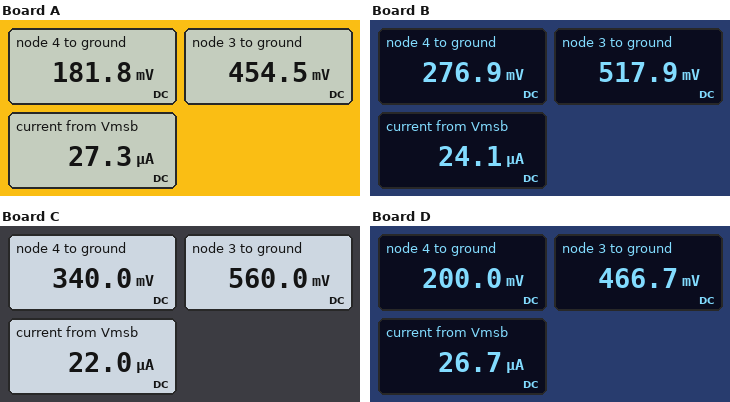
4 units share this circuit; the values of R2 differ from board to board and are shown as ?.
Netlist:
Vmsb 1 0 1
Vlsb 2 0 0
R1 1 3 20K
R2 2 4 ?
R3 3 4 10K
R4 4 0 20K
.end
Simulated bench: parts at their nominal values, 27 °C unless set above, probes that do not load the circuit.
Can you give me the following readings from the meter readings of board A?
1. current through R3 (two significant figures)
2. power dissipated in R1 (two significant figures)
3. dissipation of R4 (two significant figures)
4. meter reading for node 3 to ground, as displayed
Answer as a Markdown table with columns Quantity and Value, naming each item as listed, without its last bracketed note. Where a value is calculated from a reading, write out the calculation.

| Quantity | Value |
|---|---|
| current through R3 | (454.5 mV - 181.8 mV) / 10 kΩ = 27 µA |
| power dissipated in R1 | (1 V - 454.5 mV)^2 / 20 kΩ = 15 µW |
| dissipation of R4 | (181.8 mV)^2 / 20 kΩ = 1.7 µW |
| meter reading for node 3 to ground, as displayed | 454.5 mV |
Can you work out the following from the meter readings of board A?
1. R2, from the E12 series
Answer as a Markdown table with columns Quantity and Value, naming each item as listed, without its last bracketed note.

| Quantity | Value |
|---|---|
| R2, from the E12 series | 10 kΩ |
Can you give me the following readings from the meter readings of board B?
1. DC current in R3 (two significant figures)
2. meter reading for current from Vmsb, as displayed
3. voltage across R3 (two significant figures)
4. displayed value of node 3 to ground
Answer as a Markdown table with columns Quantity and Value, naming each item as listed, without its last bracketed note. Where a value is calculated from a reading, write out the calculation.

| Quantity | Value |
|---|---|
| DC current in R3 | (517.9 mV - 276.9 mV) / 10 kΩ = 24 µA |
| meter reading for current from Vmsb, as displayed | 24.1 µA |
| voltage across R3 | 517.9 mV - 276.9 mV = 240 mV |
| displayed value of node 3 to ground | 517.9 mV |
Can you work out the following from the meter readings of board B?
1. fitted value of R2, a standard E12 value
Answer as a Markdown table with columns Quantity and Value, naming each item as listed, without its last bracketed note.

| Quantity | Value |
|---|---|
| fitted value of R2, a standard E12 value | 27 kΩ |
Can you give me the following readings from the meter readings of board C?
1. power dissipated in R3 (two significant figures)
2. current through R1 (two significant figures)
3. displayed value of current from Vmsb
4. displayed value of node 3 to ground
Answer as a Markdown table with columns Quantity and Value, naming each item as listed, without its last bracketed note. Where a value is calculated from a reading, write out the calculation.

| Quantity | Value |
|---|---|
| power dissipated in R3 | (560 mV - 340 mV)^2 / 10 kΩ = 4.8 µW |
| current through R1 | (1 V - 560 mV) / 20 kΩ = 22 µA |
| displayed value of current from Vmsb | 22.0 µA |
| displayed value of node 3 to ground | 560.0 mV |
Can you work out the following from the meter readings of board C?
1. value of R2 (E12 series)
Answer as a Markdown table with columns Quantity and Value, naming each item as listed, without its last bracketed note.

| Quantity | Value |
|---|---|
| value of R2 | 68 kΩ |
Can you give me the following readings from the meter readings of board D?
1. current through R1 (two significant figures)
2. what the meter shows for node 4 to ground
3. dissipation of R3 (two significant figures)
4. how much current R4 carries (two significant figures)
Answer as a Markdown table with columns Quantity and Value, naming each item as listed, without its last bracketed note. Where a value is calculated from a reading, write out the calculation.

| Quantity | Value |
|---|---|
| current through R1 | (1 V - 466.7 mV) / 20 kΩ = 27 µA |
| what the meter shows for node 4 to ground | 200.0 mV |
| dissipation of R3 | (466.7 mV - 200 mV)^2 / 10 kΩ = 7.1 µW |
| how much current R4 carries | (200 mV) / 20 kΩ = 10 µA |
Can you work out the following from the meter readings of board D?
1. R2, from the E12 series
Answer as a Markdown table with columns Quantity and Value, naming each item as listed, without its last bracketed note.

| Quantity | Value |
|---|---|
| R2, from the E12 series | 12 kΩ |
